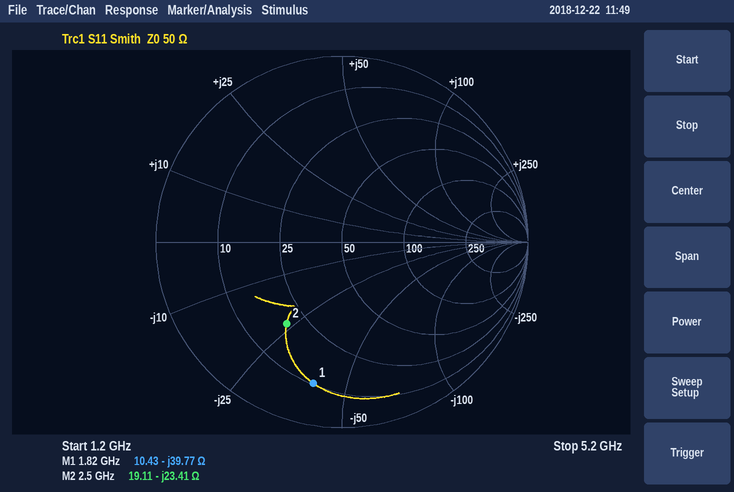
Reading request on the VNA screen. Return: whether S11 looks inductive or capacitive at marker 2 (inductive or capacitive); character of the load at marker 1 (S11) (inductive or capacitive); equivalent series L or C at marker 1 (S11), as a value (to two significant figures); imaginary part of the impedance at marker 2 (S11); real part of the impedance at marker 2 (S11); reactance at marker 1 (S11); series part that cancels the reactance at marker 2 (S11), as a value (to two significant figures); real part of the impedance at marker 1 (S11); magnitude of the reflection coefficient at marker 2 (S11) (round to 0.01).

capacitive
capacitive
2.2 pF
-23.41 Ω
19.11 Ω
-39.77 Ω
1.5 nH
10.43 Ω
0.53
